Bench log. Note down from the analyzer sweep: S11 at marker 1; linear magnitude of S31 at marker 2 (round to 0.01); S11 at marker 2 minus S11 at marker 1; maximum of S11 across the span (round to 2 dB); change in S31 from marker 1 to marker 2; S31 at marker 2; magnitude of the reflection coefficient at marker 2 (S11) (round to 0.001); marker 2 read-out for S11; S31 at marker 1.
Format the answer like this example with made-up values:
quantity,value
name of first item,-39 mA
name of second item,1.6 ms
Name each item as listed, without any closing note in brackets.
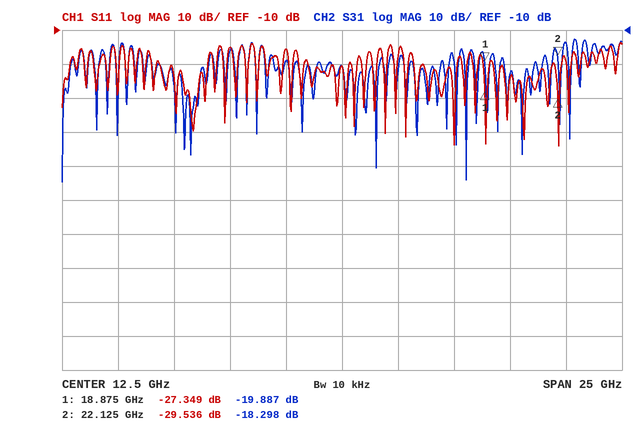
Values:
quantity,value
S11 at marker 1,-27.349 dB
linear magnitude of S31 at marker 2,0.12
S11 at marker 2 minus S11 at marker 1,-2.187 dB
maximum of S11 across the span,-14 dB
change in S31 from marker 1 to marker 2,1.589 dB
S31 at marker 2,-18.298 dB
magnitude of the reflection coefficient at marker 2 (S11),0.033
marker 2 read-out for S11,-29.536 dB
S31 at marker 1,-19.887 dB
